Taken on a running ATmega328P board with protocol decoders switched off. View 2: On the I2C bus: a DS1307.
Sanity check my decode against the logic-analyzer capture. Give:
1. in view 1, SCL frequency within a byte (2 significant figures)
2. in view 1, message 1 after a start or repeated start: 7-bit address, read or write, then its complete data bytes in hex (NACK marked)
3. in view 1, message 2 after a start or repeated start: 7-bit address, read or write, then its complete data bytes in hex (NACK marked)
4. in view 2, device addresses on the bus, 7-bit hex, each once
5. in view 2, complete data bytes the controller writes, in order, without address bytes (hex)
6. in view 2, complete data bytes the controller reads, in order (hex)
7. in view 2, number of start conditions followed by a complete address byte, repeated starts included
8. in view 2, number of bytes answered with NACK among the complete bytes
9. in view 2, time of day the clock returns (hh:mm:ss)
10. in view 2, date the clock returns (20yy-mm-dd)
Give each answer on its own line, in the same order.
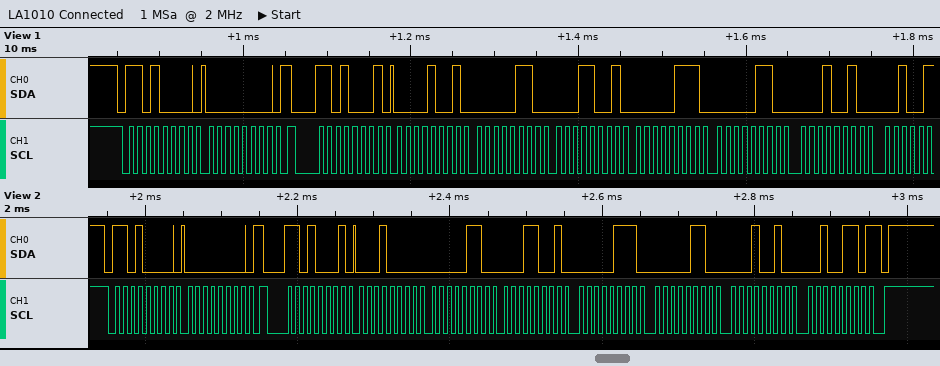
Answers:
100 kHz
0x68 write: 00
0x68 read: 09 06 19 07 06 12
0x68
00
10 06 19 07 06 12 26
2
1
19:06:10
2026-12-06
